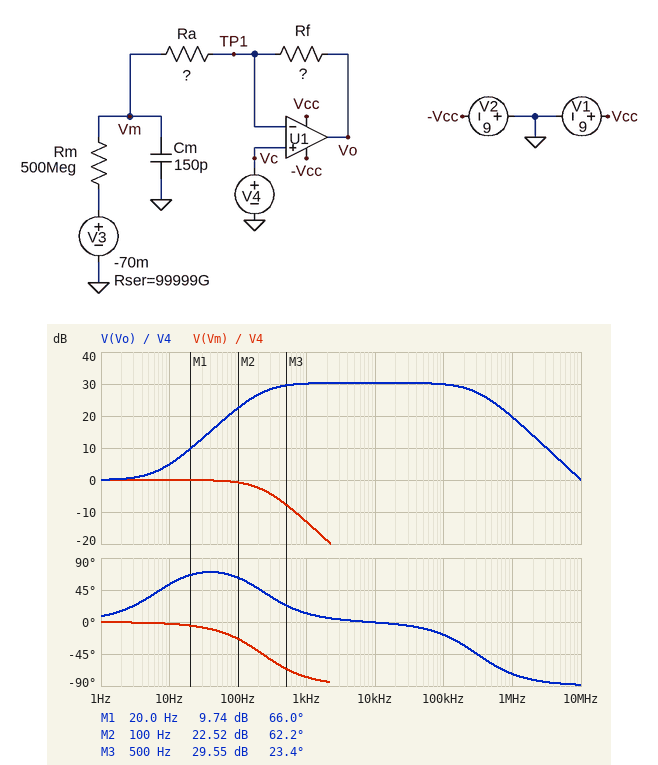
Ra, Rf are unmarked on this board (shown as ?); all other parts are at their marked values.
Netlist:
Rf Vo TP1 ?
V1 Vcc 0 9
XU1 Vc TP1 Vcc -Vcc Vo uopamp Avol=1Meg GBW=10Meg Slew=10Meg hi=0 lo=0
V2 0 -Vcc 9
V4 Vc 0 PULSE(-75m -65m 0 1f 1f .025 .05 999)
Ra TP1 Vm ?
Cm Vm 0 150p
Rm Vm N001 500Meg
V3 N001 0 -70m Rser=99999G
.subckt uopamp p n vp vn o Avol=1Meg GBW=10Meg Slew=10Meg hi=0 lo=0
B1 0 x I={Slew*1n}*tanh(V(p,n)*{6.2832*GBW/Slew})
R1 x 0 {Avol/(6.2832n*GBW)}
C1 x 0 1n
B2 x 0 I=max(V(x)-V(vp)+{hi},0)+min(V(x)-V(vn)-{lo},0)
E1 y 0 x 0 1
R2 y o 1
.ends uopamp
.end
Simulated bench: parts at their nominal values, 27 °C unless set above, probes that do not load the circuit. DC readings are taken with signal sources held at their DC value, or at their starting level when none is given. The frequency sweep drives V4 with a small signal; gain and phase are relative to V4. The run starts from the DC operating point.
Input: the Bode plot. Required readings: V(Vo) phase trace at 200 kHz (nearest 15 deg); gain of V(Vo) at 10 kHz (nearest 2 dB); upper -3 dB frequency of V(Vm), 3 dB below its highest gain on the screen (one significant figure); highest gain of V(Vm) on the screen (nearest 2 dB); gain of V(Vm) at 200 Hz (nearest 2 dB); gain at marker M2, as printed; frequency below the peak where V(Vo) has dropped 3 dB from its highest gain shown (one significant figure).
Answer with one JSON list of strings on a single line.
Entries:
["-30 deg", "30 dB", "200 Hz", "0 dB", "-2 dB", "22.52 dB", "200 Hz"]
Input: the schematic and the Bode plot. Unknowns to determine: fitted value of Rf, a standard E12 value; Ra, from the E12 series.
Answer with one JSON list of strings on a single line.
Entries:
["150 MΩ", "4.7 MΩ"]
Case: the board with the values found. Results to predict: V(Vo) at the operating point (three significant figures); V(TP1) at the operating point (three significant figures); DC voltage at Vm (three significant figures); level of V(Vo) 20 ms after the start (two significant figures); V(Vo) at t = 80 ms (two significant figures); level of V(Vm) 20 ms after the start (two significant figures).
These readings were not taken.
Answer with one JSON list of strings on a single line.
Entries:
["-75.0 mV", "-75.0 mV", "-75.0 mV", "-65 mV", "-75 mV", "-65 mV"]
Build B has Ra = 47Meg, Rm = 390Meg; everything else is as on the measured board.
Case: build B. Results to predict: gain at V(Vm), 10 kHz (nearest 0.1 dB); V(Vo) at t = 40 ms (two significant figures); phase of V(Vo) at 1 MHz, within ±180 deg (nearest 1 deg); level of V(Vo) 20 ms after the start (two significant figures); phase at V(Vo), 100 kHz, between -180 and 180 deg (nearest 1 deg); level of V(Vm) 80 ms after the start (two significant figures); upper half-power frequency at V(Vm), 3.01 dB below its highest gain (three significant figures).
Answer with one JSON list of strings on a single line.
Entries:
["-52.9 dB", "-79 mV", "-23 deg", "-63 mV", "-2 deg", "-70 mV", "22.6 Hz"]
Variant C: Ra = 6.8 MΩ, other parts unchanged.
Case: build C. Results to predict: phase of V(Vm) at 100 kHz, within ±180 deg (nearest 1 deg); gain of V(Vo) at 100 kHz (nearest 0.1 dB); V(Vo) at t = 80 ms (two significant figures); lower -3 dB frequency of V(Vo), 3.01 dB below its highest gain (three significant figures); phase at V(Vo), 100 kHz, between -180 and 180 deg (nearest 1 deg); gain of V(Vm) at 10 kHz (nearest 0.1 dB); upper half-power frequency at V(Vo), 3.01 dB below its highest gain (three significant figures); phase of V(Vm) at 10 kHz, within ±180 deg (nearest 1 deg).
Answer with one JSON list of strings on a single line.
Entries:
["-103 deg", "27.0 dB", "-77 mV", "156 Hz", "-13 deg", "-36.1 dB", "434 kHz", "-90 deg"]
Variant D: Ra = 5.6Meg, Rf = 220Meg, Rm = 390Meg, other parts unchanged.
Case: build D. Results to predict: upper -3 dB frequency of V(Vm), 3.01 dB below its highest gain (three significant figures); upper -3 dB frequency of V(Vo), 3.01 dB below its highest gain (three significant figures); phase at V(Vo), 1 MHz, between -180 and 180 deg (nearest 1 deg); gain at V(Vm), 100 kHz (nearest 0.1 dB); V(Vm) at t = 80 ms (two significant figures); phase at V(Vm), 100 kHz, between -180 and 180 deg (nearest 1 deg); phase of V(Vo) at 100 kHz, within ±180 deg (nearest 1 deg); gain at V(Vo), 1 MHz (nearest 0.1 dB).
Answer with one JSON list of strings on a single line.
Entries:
["190 Hz", "248 kHz", "-76 deg", "-55.1 dB", "-75 mV", "-112 deg", "-22 deg", "19.7 dB"]
